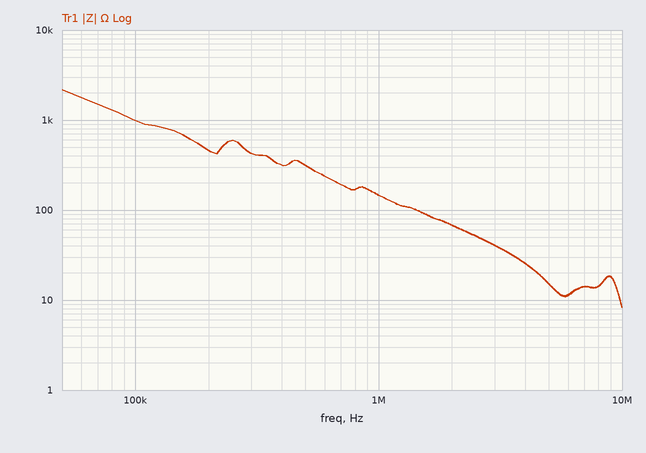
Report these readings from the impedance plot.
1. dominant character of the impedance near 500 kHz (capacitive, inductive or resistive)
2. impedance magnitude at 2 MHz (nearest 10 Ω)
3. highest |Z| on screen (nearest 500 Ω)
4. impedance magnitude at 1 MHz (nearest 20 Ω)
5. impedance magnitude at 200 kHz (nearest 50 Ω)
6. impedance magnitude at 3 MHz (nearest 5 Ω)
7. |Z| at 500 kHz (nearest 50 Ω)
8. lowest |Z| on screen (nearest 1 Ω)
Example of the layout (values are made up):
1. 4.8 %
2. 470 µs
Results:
1. capacitive
2. 70 Ω
3. 2.0 kΩ
4. 140 Ω
5. 450 Ω
6. 40 Ω
7. 300 Ω
8. 8 Ω
